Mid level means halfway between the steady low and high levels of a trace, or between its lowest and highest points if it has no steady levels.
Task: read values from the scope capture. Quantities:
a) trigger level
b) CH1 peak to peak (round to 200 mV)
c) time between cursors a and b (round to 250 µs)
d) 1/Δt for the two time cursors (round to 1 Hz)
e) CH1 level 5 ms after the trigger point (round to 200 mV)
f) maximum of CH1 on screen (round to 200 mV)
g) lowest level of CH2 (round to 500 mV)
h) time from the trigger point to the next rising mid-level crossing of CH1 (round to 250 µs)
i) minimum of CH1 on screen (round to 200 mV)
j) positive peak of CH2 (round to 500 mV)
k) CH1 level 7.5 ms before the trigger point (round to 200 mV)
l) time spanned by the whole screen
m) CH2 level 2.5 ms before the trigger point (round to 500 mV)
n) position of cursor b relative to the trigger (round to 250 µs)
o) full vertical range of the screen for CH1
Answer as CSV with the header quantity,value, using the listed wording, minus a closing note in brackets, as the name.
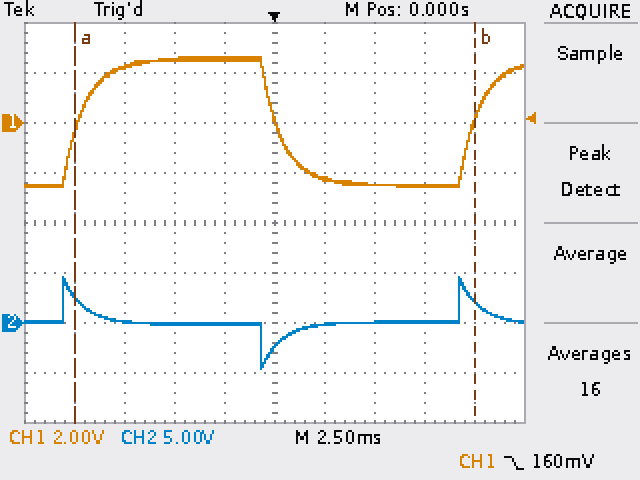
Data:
quantity,value
trigger level,160 mV
CH1 peak to peak,5.2 V
time between cursors a and b,20.00 ms
1/Δt for the two time cursors,50 Hz
CH1 level 5 ms after the trigger point,-2.4 V
maximum of CH1 on screen,2.6 V
lowest level of CH2,-4.5 V
time from the trigger point to the next rising mid-level crossing of CH1,10.00 ms
minimum of CH1 on screen,-2.6 V
positive peak of CH2,4.5 V
CH1 level 7.5 ms before the trigger point,2.2 V
time spanned by the whole screen,25 ms
CH2 level 2.5 ms before the trigger point,0.0 V
position of cursor b relative to the trigger,+10.00 ms
full vertical range of the screen for CH1,16 V
